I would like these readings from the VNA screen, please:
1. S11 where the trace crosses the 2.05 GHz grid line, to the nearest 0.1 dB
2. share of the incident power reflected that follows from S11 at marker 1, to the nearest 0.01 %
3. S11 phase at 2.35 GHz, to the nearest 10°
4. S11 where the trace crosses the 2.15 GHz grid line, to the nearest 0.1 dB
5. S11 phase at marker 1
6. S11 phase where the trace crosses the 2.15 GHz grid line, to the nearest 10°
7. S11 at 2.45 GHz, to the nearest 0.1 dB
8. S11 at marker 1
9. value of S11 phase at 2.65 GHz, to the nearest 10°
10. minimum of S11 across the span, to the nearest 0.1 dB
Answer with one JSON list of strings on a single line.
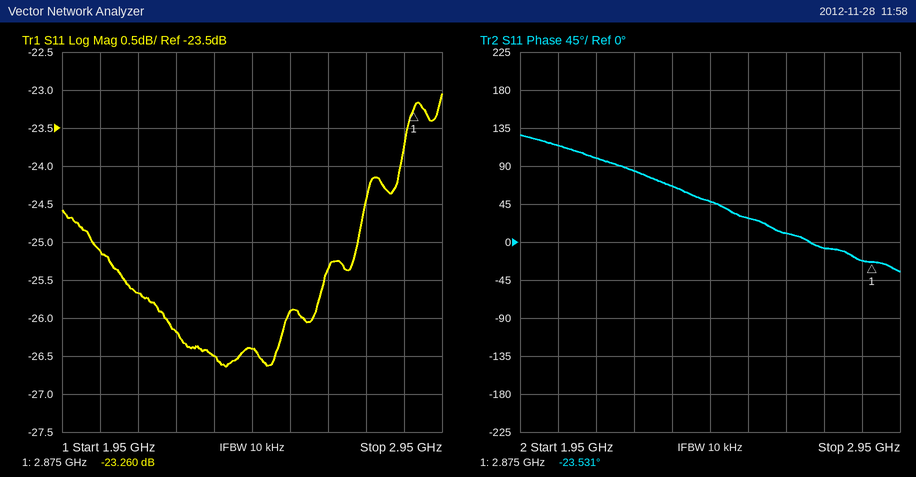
["-25.1 dB", "0.47 %", "70°", "-25.7 dB", "-23.531°", "100°", "-26.4 dB", "-23.260 dB", "10°", "-26.6 dB"]
